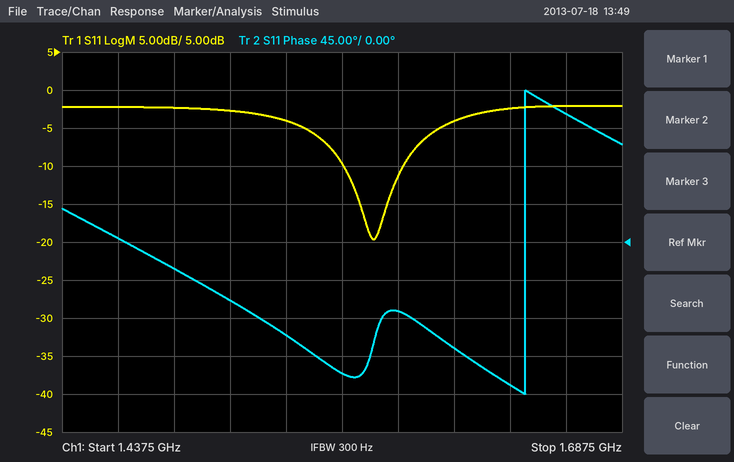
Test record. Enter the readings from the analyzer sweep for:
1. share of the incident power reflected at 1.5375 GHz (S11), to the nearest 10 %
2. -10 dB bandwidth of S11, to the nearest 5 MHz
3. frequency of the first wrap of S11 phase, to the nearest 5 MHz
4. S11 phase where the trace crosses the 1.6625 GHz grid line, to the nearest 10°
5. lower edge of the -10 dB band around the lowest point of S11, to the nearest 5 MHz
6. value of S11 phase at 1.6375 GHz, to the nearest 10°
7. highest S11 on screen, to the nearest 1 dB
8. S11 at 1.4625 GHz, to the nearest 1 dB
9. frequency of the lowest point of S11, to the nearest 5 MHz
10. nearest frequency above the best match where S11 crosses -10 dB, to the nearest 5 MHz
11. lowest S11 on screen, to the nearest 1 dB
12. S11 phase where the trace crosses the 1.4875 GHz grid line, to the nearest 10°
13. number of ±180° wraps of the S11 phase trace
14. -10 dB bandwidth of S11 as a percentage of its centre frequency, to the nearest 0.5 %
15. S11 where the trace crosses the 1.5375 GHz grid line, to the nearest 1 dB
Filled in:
40 %
25 MHz
1.645 GHz
150°
1.565 GHz
-170°
-2 dB
-2 dB
1.575 GHz
1.590 GHz
-20 dB
-30°
1
1.5 %
-4 dB
